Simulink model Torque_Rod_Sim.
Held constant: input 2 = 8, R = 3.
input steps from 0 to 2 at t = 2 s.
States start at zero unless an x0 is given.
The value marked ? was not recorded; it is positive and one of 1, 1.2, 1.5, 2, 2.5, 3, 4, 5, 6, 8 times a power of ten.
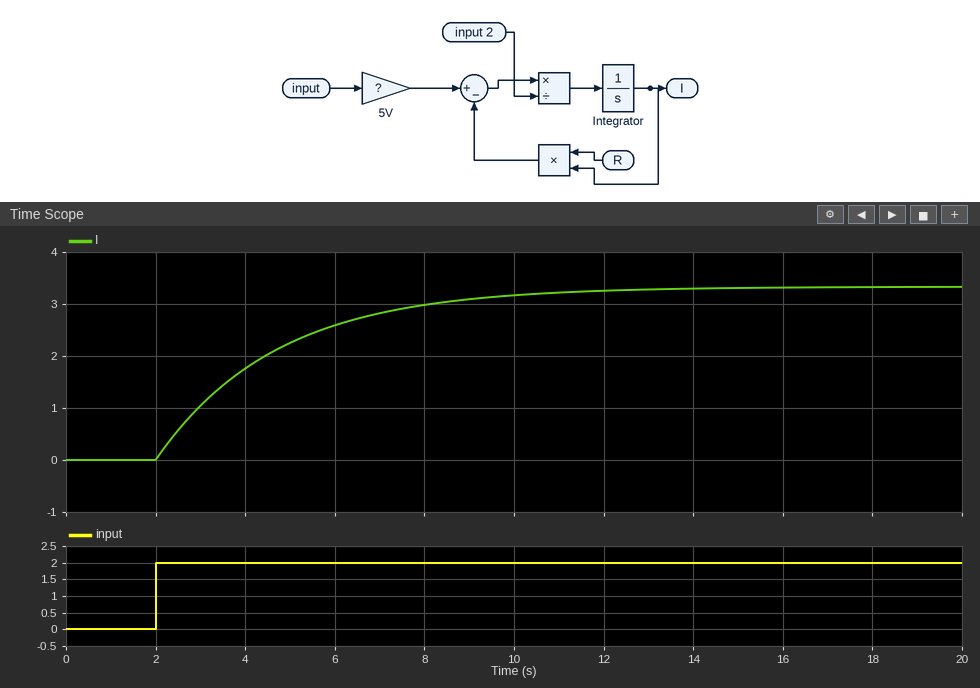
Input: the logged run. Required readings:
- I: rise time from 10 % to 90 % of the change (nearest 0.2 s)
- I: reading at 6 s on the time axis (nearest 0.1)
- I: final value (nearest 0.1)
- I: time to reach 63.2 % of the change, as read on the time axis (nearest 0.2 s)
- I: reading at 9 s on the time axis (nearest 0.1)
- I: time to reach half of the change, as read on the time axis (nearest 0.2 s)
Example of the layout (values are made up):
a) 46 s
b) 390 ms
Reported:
a) 5.8 s
b) 2.6
c) 3.3
d) 4.6 s
e) 3.1
f) 3.8 s
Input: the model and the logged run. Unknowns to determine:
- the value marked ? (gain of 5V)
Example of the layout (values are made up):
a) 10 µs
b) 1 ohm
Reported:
a) 5
